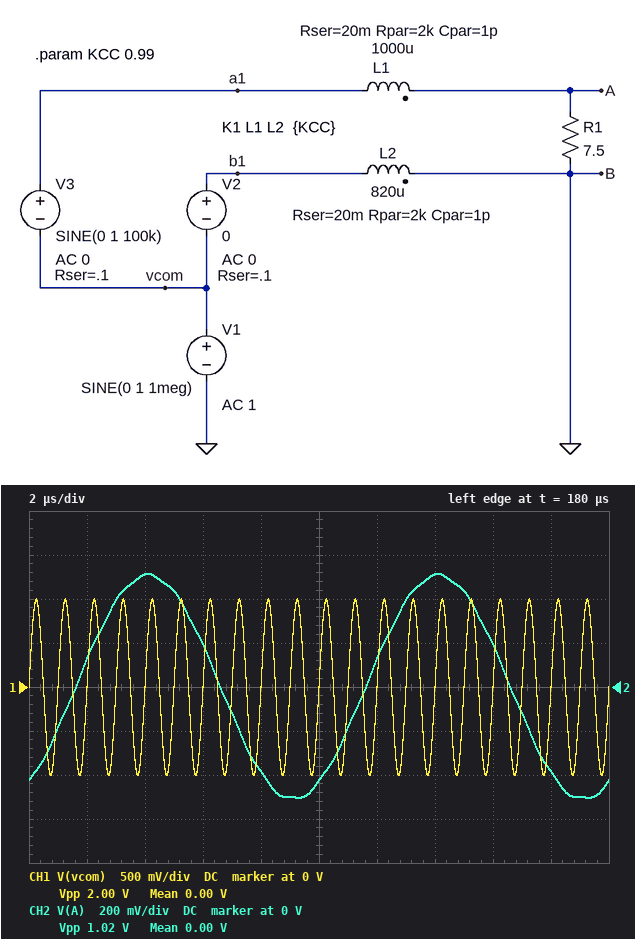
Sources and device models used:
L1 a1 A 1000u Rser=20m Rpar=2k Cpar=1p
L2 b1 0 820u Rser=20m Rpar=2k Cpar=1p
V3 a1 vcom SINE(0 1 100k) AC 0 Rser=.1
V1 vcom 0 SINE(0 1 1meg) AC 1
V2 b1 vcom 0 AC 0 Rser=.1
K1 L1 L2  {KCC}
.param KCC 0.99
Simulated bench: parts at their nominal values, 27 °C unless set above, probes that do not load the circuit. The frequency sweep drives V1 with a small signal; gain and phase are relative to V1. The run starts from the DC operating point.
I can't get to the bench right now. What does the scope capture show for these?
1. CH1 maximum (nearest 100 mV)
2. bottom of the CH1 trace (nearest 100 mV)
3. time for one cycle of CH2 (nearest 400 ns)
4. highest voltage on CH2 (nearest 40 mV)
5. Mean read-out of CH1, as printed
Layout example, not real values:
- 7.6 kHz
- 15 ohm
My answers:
- 1.0 V
- -1.0 V
- 10.0 µs
- 520 mV
- 0.00 V
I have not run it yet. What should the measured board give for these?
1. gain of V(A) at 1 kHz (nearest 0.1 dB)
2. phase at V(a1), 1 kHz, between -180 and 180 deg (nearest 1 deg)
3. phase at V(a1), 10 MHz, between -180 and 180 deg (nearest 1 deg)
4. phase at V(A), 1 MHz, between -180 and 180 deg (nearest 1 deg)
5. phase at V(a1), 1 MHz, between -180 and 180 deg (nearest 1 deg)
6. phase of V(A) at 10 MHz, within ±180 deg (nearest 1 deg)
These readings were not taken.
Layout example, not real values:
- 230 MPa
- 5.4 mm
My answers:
- -20.7 dB
- 0 deg
- 0 deg
- 60 deg
- 0 deg
- 16 deg
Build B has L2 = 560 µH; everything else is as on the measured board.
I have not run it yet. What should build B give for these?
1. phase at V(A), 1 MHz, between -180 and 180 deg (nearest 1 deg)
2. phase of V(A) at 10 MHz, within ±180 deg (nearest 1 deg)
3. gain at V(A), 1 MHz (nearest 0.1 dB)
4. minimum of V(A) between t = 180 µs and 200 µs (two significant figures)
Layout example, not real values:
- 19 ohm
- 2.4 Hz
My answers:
- 83 deg
- 33 deg
- -34.1 dB
- -510 mV
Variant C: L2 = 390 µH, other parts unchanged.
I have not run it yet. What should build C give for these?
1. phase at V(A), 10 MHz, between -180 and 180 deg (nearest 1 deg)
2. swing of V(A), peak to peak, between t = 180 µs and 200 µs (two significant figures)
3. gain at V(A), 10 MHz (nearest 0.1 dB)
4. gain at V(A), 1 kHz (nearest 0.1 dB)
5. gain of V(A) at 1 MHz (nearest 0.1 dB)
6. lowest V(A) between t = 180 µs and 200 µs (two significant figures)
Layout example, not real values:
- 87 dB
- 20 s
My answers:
- 47 deg
- 1.1 V
- -45.3 dB
- -5.1 dB
- -29.1 dB
- -530 mV
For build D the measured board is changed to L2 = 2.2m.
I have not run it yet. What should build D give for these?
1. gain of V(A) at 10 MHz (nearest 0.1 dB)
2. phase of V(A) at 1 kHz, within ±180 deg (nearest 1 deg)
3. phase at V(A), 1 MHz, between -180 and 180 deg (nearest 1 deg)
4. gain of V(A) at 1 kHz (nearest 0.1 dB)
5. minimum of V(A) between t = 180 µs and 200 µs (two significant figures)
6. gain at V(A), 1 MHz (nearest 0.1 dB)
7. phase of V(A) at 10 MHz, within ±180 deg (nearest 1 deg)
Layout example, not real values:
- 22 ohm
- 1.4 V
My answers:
- -47.9 dB
- -2 deg
- -76 deg
- -9.8 dB
- -530 mV
- -33.9 dB
- -22 deg
